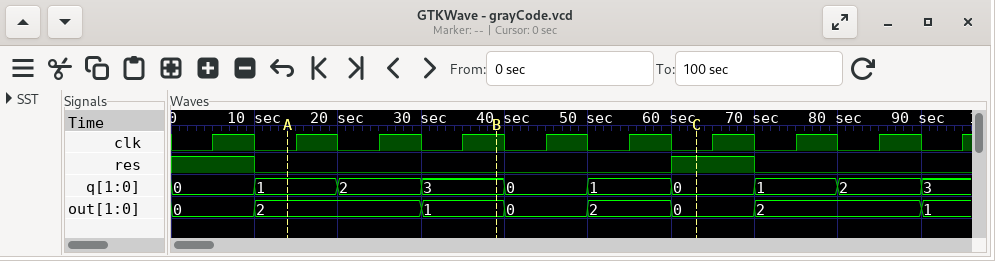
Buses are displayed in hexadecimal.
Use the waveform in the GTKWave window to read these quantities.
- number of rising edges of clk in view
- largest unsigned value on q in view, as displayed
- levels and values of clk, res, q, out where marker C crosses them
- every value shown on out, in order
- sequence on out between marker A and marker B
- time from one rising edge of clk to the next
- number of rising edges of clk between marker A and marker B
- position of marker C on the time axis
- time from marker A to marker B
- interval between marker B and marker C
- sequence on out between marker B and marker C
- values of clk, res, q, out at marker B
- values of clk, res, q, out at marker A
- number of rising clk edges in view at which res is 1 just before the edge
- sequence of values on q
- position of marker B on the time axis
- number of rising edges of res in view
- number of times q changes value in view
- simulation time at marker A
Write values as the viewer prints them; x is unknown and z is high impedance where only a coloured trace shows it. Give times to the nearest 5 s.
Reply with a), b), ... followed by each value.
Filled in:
a) 10
b) 3
c) clk=0, res=1, q=0, out=0
d) 0, 2, 1, 0, 2, 0, 2, 1
e) 2, 1
f) 10 s
g) 3
h) 65 s
i) 25 s
j) 25 s
k) 1, 0, 2, 0
l) clk=1, res=0, q=3, out=1
m) clk=0, res=0, q=1, out=2
n) 2
o) 0, 1, 2, 3, 0, 1, 0, 1, 2, 3
p) 40 s
q) 1
r) 9
s) 15 s
